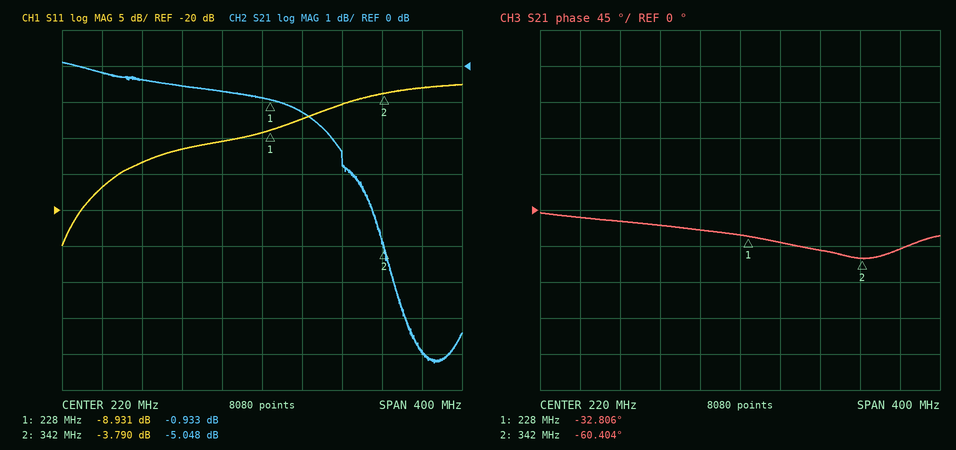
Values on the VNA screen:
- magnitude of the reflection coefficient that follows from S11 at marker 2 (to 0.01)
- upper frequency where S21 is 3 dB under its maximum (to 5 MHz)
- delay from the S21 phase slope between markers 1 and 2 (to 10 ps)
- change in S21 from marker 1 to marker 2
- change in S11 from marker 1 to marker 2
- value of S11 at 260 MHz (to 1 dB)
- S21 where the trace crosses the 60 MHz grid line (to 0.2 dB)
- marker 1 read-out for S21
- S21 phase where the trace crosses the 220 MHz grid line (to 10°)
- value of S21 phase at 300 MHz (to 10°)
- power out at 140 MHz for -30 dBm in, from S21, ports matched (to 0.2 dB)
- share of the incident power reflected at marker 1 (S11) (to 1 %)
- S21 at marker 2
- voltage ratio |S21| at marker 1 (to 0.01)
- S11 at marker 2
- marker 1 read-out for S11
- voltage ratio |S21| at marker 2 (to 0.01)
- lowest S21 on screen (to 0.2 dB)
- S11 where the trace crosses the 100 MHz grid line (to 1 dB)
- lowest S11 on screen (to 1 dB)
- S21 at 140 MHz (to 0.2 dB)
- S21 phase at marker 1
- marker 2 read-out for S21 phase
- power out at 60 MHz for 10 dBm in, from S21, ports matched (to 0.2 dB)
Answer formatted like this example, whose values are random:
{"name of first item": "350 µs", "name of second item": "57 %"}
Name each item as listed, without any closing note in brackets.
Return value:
{"magnitude of the reflection coefficient that follows from S11 at marker 2": "0.65", "upper frequency where S21 is 3 dB under its maximum": "305 MHz", "delay from the S21 phase slope between markers 1 and 2": "670 ps", "change in S21 from marker 1 to marker 2": "-4.115 dB", "change in S11 from marker 1 to marker 2": "5.141 dB", "value of S11 at 260 MHz": "-7 dB", "S21 where the trace crosses the 60 MHz grid line": "-0.2 dB", "marker 1 read-out for S21": "-0.933 dB", "S21 phase where the trace crosses the 220 MHz grid line": "-30°", "value of S21 phase at 300 MHz": "-50°", "power out at 140 MHz for -30 dBm in, from S21, ports matched": "-30.6 dBm", "share of the incident power reflected at marker 1 (S11)": "13 %", "S21 at marker 2": "-5.048 dB", "voltage ratio |S21| at marker 1": "0.90", "S11 at marker 2": "-3.790 dB", "marker 1 read-out for S11": "-8.931 dB", "voltage ratio |S21| at marker 2": "0.56", "lowest S21 on screen": "-8.2 dB", "S11 where the trace crosses the 100 MHz grid line": "-13 dB", "lowest S11 on screen": "-25 dB", "S21 at 140 MHz": "-0.6 dB", "S21 phase at marker 1": "-32.806°", "marker 2 read-out for S21 phase": "-60.404°", "power out at 60 MHz for 10 dBm in, from S21, ports matched": "9.8 dBm"}
